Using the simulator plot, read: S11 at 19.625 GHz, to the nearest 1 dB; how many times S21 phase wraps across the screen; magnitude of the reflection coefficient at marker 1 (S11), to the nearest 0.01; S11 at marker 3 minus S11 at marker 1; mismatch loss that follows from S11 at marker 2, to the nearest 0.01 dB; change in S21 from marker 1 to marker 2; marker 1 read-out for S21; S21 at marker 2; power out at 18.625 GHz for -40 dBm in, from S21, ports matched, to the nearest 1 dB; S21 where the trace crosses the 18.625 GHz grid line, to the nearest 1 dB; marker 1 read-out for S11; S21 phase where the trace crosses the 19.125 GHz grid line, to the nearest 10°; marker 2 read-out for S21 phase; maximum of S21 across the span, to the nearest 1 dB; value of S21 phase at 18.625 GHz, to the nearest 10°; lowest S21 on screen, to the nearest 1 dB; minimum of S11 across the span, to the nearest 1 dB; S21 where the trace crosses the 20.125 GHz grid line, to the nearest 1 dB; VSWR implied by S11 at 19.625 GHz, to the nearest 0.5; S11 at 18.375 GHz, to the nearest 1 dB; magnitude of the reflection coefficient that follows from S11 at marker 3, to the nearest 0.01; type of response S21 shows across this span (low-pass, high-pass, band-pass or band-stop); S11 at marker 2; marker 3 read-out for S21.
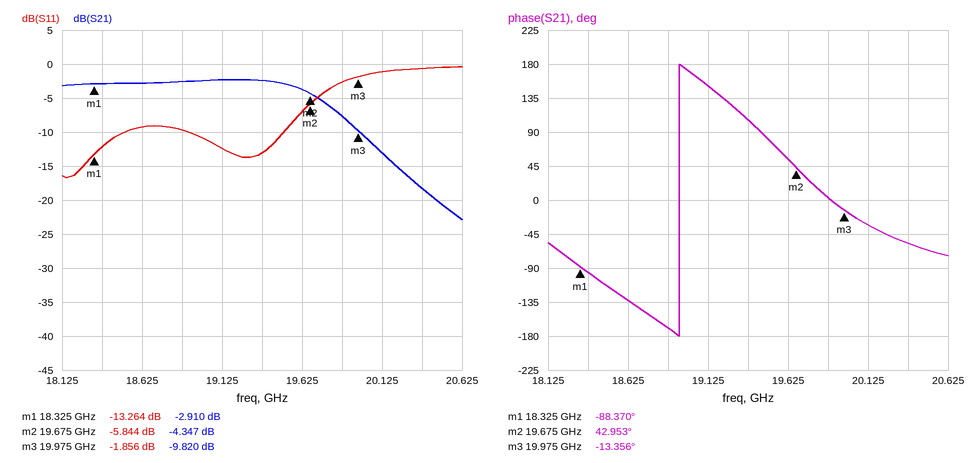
-7 dB
1
0.22
11.408 dB
1.31 dB
-1.437 dB
-2.910 dB
-4.347 dB
-43 dBm
-3 dB
-13.264 dB
150°
42.953°
-2 dB
-130°
-23 dB
-17 dB
-13 dB
2.5
-12 dB
0.81
low-pass
-5.844 dB
-9.820 dB
